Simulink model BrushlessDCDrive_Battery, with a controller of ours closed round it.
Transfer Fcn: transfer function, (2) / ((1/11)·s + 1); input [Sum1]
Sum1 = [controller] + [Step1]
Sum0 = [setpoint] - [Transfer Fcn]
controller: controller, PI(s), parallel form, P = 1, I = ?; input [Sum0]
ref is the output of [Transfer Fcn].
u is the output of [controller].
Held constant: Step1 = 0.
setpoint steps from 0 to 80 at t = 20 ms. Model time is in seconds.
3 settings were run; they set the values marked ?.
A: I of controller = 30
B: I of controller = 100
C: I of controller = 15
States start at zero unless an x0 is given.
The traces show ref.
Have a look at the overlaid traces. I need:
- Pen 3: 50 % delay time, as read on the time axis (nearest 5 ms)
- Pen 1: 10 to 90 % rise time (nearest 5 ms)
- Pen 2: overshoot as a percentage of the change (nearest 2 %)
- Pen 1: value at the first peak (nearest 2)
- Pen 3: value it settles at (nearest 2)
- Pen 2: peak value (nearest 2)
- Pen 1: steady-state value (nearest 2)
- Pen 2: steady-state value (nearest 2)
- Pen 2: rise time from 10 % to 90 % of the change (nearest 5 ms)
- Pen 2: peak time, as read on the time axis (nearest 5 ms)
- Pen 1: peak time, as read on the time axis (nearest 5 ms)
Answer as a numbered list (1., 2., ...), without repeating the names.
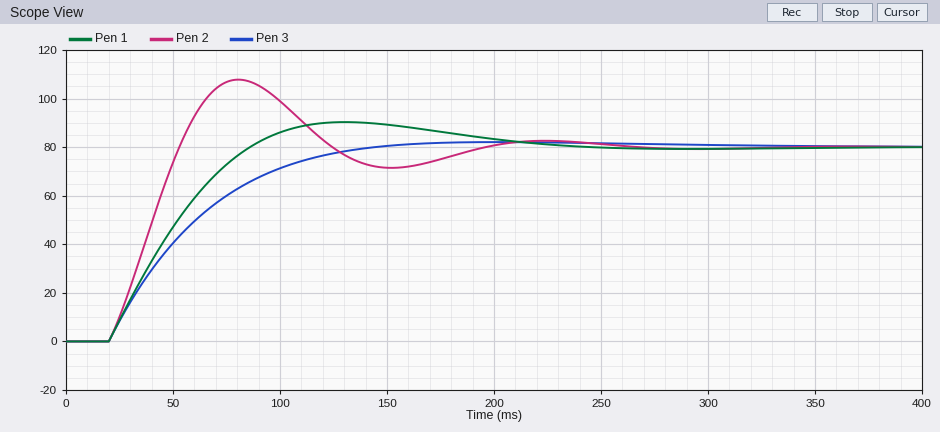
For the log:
1. 50 ms
2. 50 ms
3. 34 %
4. 90
5. 80
6. 108
7. 80
8. 80
9. 25 ms
10. 80 ms
11. 130 ms
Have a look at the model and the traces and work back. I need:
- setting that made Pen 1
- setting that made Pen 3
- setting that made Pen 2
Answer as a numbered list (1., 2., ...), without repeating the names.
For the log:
1. A
2. C
3. B
